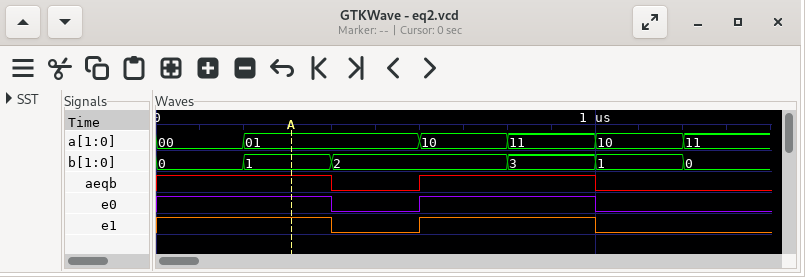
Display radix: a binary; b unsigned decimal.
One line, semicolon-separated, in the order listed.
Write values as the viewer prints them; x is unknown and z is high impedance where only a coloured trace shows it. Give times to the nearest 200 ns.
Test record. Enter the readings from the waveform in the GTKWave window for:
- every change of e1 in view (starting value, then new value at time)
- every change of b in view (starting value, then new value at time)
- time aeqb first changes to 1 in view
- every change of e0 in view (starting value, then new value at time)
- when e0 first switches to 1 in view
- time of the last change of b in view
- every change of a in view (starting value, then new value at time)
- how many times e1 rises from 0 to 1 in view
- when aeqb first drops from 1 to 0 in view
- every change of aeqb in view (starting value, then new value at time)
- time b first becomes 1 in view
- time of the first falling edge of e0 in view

1, 0 at 400 ns, 1 at 600 ns, 0 at 1000 ns; 0, 1 at 200 ns, 2 at 400 ns, 3 at 800 ns, 1 at 1000 ns, 0 at 1200 ns; 600 ns; 1, 0 at 400 ns, 1 at 600 ns, 0 at 1000 ns; 600 ns; 1200 ns; 00, 01 at 200 ns, 10 at 600 ns, 11 at 800 ns, 10 at 1000 ns, 11 at 1200 ns; 1; 400 ns; 1, 0 at 400 ns, 1 at 600 ns, 0 at 1000 ns; 200 ns; 400 ns
